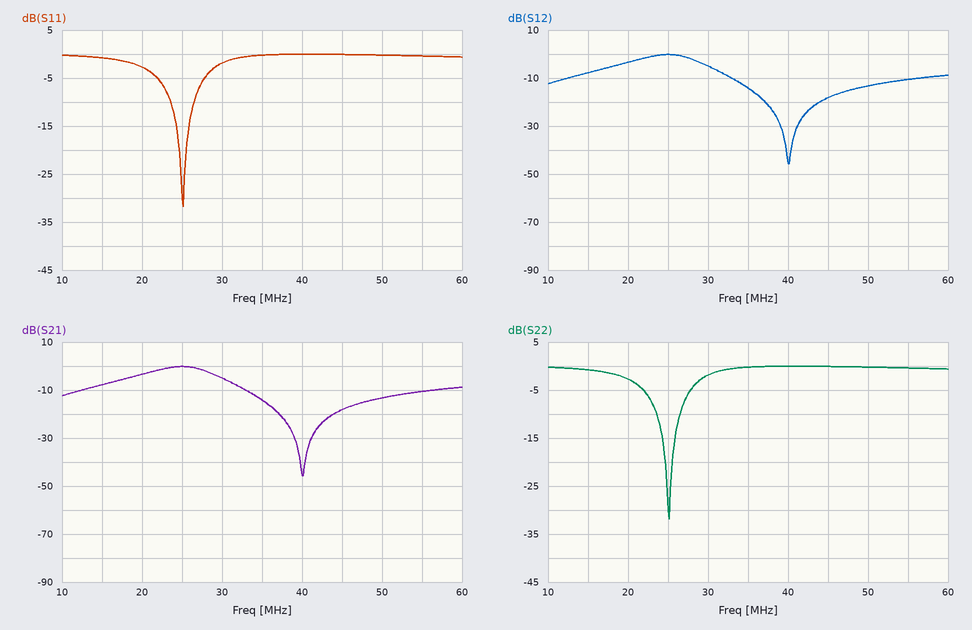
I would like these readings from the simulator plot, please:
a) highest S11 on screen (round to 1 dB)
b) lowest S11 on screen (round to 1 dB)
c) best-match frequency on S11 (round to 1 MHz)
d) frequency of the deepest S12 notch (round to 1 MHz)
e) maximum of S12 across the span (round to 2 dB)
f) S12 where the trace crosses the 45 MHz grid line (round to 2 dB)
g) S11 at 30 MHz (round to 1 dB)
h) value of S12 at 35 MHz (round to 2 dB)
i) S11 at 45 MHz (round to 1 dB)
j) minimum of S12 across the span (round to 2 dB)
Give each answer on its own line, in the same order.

0 dB
-32 dB
25 MHz
40 MHz
0 dB
-18 dB
-2 dB
-14 dB
0 dB
-46 dB
